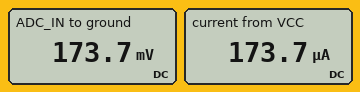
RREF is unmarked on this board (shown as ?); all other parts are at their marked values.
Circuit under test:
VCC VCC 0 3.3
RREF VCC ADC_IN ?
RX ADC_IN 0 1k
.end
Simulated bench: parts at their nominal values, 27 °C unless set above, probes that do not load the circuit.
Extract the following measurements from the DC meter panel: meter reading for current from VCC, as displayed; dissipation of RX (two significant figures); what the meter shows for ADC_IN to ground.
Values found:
173.7 µA
30 µW
173.7 mV
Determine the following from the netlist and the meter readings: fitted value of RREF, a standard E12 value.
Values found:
18 kΩ
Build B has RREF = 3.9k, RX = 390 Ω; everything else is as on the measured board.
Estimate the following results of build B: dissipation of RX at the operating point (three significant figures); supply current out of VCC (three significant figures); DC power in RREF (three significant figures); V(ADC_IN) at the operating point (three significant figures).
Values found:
231 µW
769 µA
2.31 mW
300 mV
